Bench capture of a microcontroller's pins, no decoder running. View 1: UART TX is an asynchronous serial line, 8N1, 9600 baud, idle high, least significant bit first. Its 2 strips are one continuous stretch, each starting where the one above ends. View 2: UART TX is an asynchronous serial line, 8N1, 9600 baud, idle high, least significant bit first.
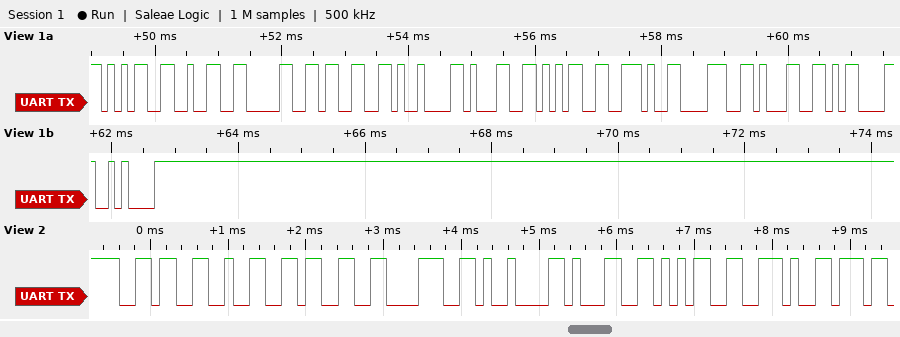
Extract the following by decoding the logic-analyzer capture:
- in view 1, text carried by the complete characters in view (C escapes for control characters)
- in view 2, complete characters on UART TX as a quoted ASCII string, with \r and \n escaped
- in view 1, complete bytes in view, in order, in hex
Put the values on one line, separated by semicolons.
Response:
"5203\t15.81\r\n"; "6238\t15."; 35 32 30 33 09 31 35 2E 38 31 0D 0A
